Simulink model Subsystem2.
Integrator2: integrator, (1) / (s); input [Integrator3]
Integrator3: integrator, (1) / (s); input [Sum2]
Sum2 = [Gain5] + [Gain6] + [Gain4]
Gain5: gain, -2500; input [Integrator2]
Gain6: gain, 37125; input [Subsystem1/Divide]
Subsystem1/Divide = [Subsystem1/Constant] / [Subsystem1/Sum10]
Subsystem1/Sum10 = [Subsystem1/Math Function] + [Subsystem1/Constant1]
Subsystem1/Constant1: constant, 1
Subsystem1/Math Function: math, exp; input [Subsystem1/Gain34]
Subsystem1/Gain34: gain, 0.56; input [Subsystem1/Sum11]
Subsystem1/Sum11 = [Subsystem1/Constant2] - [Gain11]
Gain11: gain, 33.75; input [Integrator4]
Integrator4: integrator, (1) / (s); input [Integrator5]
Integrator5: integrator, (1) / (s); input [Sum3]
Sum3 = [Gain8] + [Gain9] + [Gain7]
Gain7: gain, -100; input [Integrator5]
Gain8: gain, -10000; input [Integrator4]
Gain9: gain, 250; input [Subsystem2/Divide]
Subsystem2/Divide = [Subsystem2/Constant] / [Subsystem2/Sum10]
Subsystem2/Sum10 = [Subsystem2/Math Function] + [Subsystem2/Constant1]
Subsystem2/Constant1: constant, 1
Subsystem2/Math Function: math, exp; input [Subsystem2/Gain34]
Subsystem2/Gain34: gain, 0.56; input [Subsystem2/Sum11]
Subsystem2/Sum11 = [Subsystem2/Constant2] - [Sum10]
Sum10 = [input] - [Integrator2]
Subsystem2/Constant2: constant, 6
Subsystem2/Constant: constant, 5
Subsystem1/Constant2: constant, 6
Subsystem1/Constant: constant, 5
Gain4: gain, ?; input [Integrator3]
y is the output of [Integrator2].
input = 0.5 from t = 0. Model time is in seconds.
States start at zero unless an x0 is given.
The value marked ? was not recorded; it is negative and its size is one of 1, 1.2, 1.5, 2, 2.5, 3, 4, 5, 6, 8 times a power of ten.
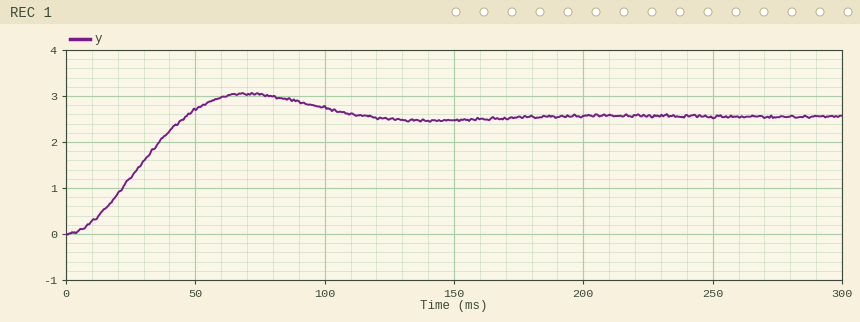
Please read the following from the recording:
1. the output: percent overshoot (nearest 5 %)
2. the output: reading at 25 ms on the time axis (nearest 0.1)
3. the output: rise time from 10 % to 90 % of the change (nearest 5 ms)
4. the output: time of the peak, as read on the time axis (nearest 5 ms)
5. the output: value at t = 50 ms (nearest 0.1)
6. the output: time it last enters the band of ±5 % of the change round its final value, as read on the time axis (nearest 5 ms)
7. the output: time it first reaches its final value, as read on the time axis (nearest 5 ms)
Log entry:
20 %
1.2
30 ms
70 ms
2.7
105 ms
45 ms
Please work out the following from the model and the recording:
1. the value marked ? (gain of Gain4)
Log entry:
-50
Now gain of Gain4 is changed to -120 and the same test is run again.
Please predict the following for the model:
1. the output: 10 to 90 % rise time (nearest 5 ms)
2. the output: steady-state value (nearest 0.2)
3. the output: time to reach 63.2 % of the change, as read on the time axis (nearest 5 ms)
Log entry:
80 ms
2.6
45 ms
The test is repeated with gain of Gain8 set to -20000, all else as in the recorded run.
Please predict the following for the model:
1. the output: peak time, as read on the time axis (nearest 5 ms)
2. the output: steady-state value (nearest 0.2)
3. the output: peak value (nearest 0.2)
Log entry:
70 ms
2.6
3.0
